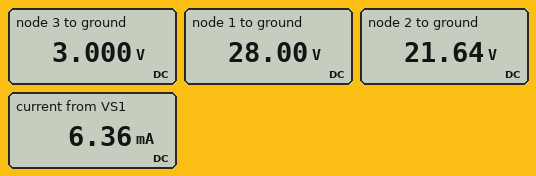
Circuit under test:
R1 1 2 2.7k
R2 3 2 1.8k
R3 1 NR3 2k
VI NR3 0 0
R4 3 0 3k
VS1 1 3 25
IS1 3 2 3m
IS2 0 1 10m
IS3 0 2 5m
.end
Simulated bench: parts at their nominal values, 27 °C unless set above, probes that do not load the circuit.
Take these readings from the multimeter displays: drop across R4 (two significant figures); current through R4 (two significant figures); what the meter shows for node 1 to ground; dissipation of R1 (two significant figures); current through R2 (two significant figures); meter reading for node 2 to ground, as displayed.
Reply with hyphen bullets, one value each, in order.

- 3.0 V
- 1.0 mA
- 28.00 V
- 15 mW
- 10 mA
- 21.64 V
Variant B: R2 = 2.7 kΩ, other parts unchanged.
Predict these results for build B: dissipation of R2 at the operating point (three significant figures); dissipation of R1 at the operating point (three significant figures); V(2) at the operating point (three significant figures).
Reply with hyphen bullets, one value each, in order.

- 201 mW
- 1.07 mW
- 26.3 V
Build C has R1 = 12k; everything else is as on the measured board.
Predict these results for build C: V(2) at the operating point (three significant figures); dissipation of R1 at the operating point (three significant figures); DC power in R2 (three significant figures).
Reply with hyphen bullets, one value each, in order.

- 18.8 V
- 7.08 mW
- 138 mW
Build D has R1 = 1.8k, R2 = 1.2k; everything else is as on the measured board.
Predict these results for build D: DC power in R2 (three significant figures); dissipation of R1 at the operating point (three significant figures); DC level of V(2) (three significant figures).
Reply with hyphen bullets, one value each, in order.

- 207 mW
- 47.4 mW
- 18.8 V
